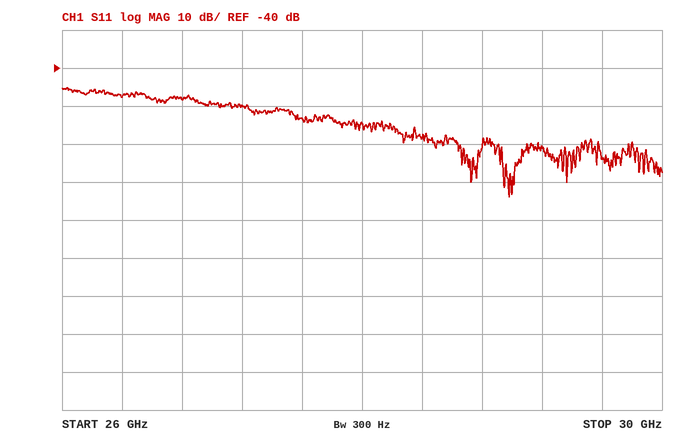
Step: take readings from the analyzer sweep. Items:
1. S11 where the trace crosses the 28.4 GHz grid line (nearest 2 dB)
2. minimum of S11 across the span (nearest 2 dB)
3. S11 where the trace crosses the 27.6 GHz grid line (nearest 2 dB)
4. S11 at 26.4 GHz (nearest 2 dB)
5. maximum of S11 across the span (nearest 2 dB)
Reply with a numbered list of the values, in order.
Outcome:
1. -58 dB
2. -74 dB
3. -54 dB
4. -48 dB
5. -46 dB
